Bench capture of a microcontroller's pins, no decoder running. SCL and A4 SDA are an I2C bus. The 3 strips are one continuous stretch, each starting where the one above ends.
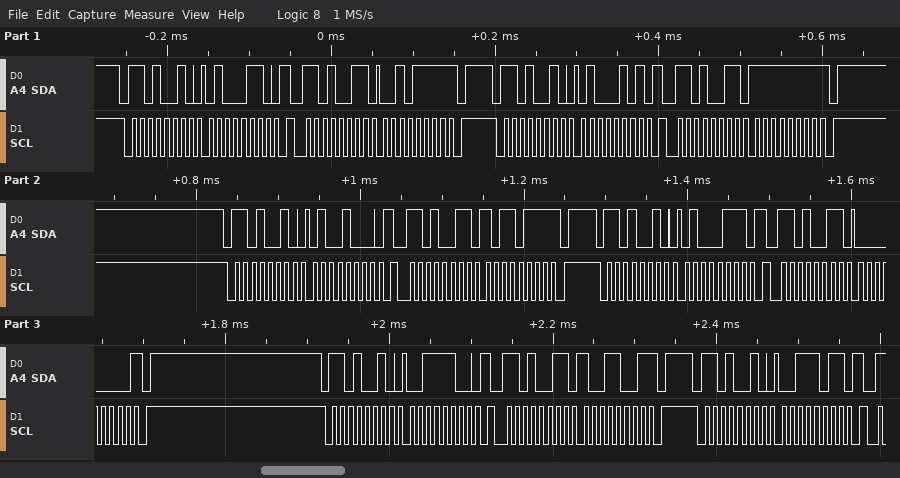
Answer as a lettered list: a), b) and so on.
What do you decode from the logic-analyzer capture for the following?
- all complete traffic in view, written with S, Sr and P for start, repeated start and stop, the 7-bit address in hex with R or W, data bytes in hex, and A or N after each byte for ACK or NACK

a) S 69W A 46 A Sr 69R A 2F N P S 69W A 45 A Sr 69R A FF N P S 69W A 48 A Sr 69R A B7 N P S 69W A 47 A Sr 69R A 00 N P S 69W A 3C A Sr 69R A 99 N P S 69W A 3B A
